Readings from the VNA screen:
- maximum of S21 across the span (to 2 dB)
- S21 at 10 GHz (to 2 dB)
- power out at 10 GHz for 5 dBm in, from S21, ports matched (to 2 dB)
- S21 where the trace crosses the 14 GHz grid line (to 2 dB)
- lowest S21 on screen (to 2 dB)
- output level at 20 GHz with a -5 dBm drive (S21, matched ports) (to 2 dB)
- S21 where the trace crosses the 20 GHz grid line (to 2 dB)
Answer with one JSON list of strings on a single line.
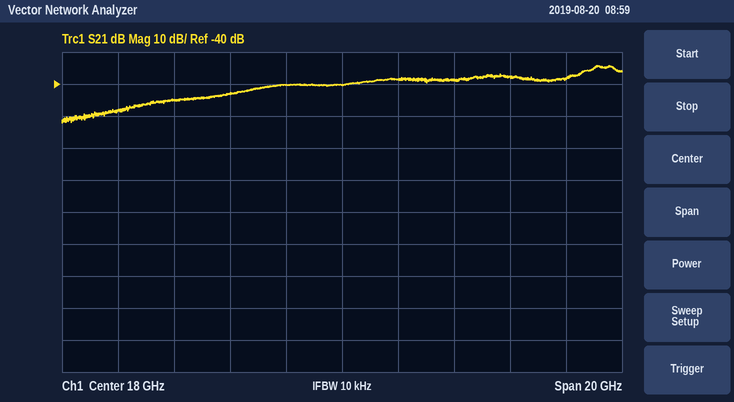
["-34 dB", "-48 dB", "-44 dBm", "-42 dB", "-52 dB", "-44 dBm", "-38 dB"]
